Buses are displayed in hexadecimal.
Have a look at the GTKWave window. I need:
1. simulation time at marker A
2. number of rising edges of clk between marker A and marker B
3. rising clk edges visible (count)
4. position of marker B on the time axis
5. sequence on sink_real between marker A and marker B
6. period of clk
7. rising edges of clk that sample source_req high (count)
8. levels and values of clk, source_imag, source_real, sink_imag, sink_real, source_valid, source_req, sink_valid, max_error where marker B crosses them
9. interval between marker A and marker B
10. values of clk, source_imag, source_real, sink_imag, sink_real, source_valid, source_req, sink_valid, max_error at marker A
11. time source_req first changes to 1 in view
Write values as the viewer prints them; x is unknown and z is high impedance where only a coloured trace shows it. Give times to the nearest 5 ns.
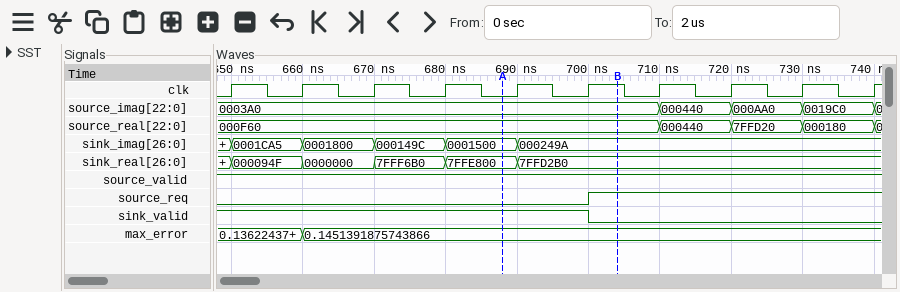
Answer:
690 ns
2
10
705 ns
7FFE800, 7FFD2B0
10 ns
4
clk=1, source_imag=0003A0, source_real=000F60, sink_imag=000249A, sink_real=7FFD2B0, source_valid=1, source_req=1, sink_valid=0, max_error=0.1451391875743866
15 ns
clk=0, source_imag=0003A0, source_real=000F60, sink_imag=0001500, sink_real=7FFE800, source_valid=1, source_req=0, sink_valid=1, max_error=0.1451391875743866
700 ns
